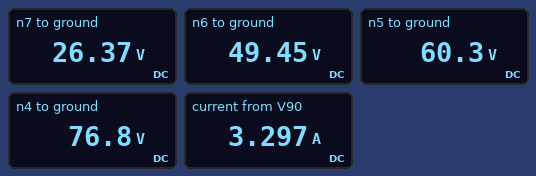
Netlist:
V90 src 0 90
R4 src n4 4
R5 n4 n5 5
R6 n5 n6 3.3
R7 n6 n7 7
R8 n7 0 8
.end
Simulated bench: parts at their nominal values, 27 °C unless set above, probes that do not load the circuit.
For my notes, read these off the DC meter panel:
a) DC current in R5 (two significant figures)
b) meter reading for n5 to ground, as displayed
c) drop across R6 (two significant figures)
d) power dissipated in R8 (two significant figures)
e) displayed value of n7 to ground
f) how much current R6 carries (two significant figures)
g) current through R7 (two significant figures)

3.3 A
60.3 V
11 V
87 W
26.37 V
3.3 A
3.3 A
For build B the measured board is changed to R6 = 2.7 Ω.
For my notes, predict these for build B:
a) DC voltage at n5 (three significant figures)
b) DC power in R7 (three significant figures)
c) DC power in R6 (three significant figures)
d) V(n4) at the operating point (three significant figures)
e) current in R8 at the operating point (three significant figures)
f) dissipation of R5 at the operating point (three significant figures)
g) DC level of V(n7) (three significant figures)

59.7 V
79.5 W
30.7 W
76.5 V
3.37 A
56.8 W
27.0 V
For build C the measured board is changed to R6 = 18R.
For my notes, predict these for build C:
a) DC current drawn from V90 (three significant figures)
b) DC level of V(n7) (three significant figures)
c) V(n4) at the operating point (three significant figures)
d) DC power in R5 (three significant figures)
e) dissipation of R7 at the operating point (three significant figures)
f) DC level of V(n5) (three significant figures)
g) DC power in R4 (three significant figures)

2.14 A
17.1 V
81.4 V
23.0 W
32.1 W
70.7 V
18.4 W
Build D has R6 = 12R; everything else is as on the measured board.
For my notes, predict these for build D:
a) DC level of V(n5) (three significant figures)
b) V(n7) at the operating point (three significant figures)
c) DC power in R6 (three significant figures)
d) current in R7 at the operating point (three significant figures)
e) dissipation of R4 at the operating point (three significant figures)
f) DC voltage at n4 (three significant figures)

67.5 V
20.0 V
75.0 W
2.50 A
25.0 W
80.0 V
